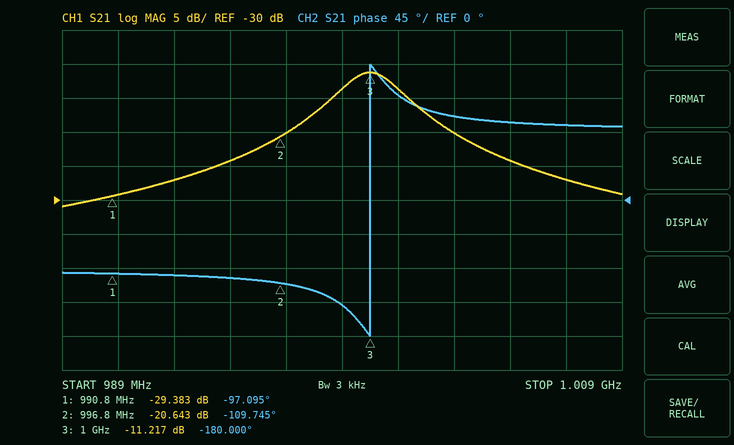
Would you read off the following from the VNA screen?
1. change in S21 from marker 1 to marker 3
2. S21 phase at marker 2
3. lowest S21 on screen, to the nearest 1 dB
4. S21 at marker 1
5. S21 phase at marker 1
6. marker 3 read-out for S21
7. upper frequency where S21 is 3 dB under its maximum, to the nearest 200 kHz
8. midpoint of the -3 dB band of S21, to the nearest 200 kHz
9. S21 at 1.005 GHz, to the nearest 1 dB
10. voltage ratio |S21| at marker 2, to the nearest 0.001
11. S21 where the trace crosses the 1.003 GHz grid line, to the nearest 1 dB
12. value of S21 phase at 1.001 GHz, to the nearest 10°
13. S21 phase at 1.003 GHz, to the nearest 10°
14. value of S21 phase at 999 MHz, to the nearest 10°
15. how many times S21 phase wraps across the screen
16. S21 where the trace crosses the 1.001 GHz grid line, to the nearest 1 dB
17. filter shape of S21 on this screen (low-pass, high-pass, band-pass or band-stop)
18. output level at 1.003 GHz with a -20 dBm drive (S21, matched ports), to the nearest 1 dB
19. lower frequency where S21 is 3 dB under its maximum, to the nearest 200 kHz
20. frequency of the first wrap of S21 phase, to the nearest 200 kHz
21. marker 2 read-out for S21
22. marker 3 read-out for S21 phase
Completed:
18.166 dB
-109.745°
-31 dB
-29.383 dB
-97.095°
-11.217 dB
1.0012 GHz
1.0000 GHz
-24 dB
0.093
-20 dB
140°
110°
-140°
1
-14 dB
band-pass
-40 dBm
998.8 MHz
1.0000 GHz
-20.643 dB
-180.000°
